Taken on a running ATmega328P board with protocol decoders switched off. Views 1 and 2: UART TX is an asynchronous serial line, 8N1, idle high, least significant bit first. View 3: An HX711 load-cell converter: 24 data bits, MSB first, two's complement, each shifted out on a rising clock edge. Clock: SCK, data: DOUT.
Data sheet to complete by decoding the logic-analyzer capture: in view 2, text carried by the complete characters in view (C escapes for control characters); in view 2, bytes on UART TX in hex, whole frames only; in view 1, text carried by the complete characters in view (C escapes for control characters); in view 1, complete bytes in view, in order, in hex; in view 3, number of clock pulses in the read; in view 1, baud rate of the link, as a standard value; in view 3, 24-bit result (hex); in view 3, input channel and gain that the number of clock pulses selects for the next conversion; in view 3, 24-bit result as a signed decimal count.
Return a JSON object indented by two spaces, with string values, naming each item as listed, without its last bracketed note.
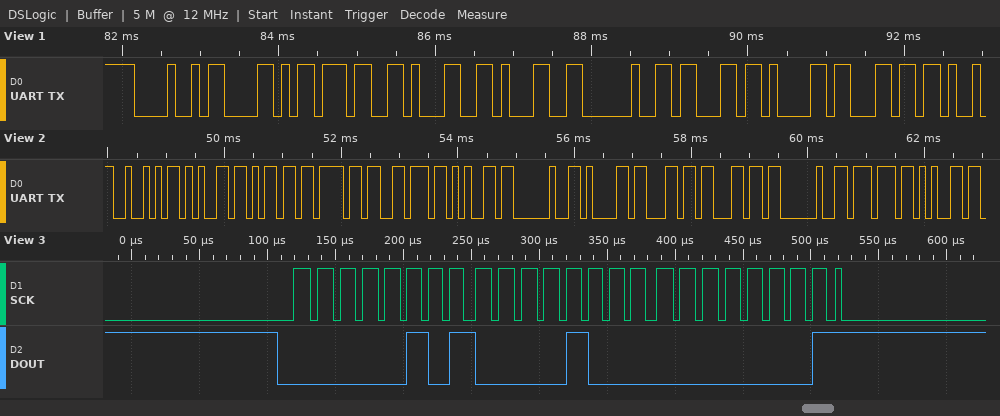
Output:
{
  "in view 2, text carried by the complete characters in view": "\"Remove all we\"",
  "in view 2, bytes on UART TX in hex, whole frames only": "52 65 6D 6F 76 65 20 61 6C 6C 20 77 65",
  "in view 1, text carried by the complete characters in view": "\"HX711 cal\"",
  "in view 1, complete bytes in view, in order, in hex": "48 58 37 31 31 20 63 61 6C",
  "in view 3, number of clock pulses in the read": "25",
  "in view 1, baud rate of the link, as a standard value": "9600 baud",
  "in view 3, 24-bit result": "0x050801",
  "in view 3, input channel and gain that the number of clock pulses selects for the next conversion": "channel A, gain 128",
  "in view 3, 24-bit result as a signed decimal count": "329729"
}
